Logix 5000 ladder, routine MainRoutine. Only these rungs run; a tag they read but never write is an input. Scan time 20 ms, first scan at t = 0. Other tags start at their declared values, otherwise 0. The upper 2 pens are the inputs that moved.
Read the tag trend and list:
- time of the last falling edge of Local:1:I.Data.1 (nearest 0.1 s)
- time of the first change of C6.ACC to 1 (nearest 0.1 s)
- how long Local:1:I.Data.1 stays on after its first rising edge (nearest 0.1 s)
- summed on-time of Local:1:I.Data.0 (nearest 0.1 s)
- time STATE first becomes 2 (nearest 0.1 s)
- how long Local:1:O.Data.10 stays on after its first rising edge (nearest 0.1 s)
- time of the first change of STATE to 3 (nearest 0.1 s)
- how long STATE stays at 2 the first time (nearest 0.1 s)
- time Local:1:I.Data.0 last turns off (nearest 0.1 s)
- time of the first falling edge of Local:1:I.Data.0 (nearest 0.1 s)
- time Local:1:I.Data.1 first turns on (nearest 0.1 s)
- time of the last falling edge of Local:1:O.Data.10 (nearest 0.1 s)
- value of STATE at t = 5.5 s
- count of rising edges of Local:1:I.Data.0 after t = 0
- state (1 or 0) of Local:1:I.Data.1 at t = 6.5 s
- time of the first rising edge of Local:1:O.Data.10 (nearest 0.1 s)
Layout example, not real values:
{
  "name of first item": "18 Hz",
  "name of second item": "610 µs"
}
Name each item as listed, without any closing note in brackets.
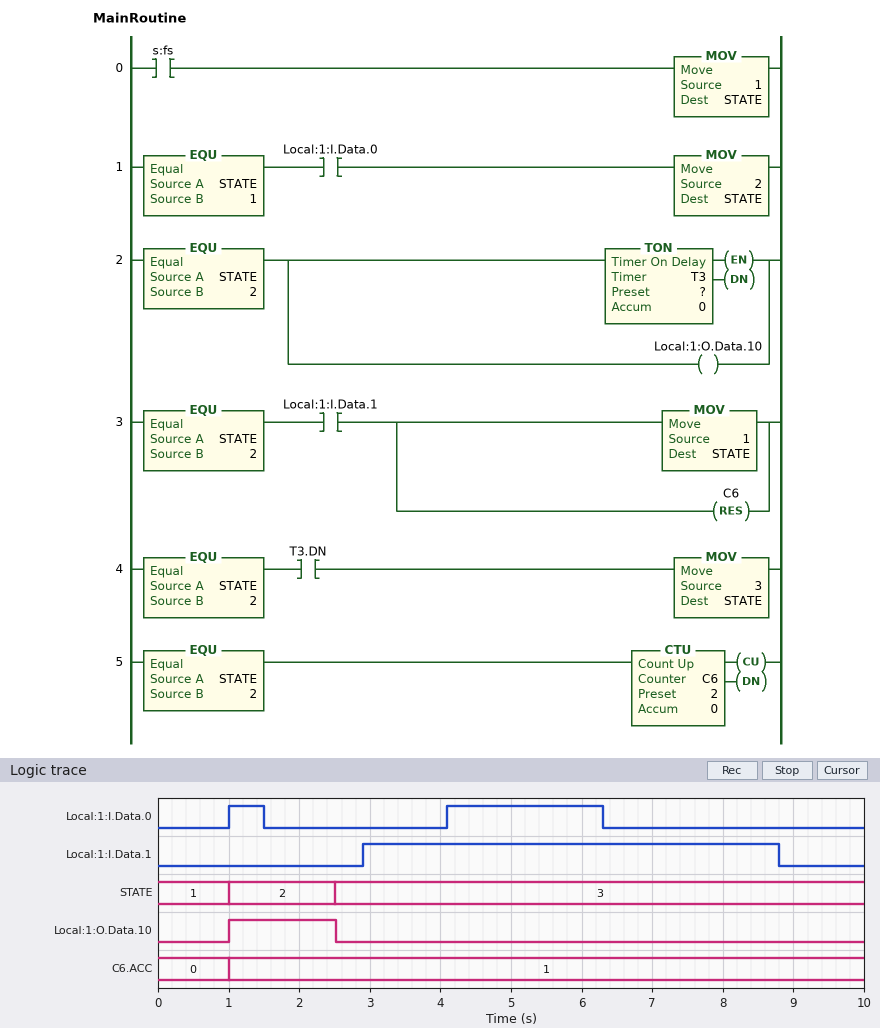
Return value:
{
  "time of the last falling edge of Local:1:I.Data.1": "8.8 s",
  "time of the first change of C6.ACC to 1": "1.0 s",
  "how long Local:1:I.Data.1 stays on after its first rising edge": "5.9 s",
  "summed on-time of Local:1:I.Data.0": "2.7 s",
  "time STATE first becomes 2": "1.0 s",
  "how long Local:1:O.Data.10 stays on after its first rising edge": "1.5 s",
  "time of the first change of STATE to 3": "2.5 s",
  "how long STATE stays at 2 the first time": "1.5 s",
  "time Local:1:I.Data.0 last turns off": "6.3 s",
  "time of the first falling edge of Local:1:I.Data.0": "1.5 s",
  "time Local:1:I.Data.1 first turns on": "2.9 s",
  "time of the last falling edge of Local:1:O.Data.10": "2.5 s",
  "value of STATE at t = 5.5 s": "3",
  "count of rising edges of Local:1:I.Data.0 after t = 0": "2",
  "state (1 or 0) of Local:1:I.Data.1 at t = 6.5 s": "1",
  "time of the first rising edge of Local:1:O.Data.10": "1.0 s"
}
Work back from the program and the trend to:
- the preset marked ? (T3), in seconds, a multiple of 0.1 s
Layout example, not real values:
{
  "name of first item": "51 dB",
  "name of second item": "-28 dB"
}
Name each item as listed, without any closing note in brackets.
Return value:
{
  "the preset marked ? (T3), in seconds, a multiple of 0.1 s": "1.5 s"
}
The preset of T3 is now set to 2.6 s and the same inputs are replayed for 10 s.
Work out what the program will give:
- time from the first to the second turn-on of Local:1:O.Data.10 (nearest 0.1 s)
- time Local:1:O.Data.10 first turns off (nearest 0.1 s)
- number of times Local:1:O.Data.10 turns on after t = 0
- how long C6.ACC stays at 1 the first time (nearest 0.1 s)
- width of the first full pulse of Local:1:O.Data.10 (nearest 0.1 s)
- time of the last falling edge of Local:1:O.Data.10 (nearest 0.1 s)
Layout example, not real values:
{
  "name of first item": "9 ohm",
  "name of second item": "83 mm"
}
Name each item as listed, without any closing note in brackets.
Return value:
{
  "time from the first to the second turn-on of Local:1:O.Data.10": "3.1 s",
  "time Local:1:O.Data.10 first turns off": "2.9 s",
  "number of times Local:1:O.Data.10 turns on after t = 0": "2",
  "how long C6.ACC stays at 1 the first time": "1.9 s",
  "width of the first full pulse of Local:1:O.Data.10": "1.9 s",
  "time of the last falling edge of Local:1:O.Data.10": "6.3 s"
}
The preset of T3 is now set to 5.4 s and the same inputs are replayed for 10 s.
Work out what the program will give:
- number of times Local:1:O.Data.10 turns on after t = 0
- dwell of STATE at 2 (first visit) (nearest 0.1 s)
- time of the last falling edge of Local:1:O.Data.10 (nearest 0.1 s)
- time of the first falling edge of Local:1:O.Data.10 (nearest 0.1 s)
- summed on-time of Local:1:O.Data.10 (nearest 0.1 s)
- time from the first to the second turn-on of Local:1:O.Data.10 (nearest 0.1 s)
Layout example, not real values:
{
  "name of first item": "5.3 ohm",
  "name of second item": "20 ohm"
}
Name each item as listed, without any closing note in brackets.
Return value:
{
  "number of times Local:1:O.Data.10 turns on after t = 0": "2",
  "dwell of STATE at 2 (first visit)": "1.9 s",
  "time of the last falling edge of Local:1:O.Data.10": "6.3 s",
  "time of the first falling edge of Local:1:O.Data.10": "2.9 s",
  "summed on-time of Local:1:O.Data.10": "4.1 s",
  "time from the first to the second turn-on of Local:1:O.Data.10": "3.1 s"
}
